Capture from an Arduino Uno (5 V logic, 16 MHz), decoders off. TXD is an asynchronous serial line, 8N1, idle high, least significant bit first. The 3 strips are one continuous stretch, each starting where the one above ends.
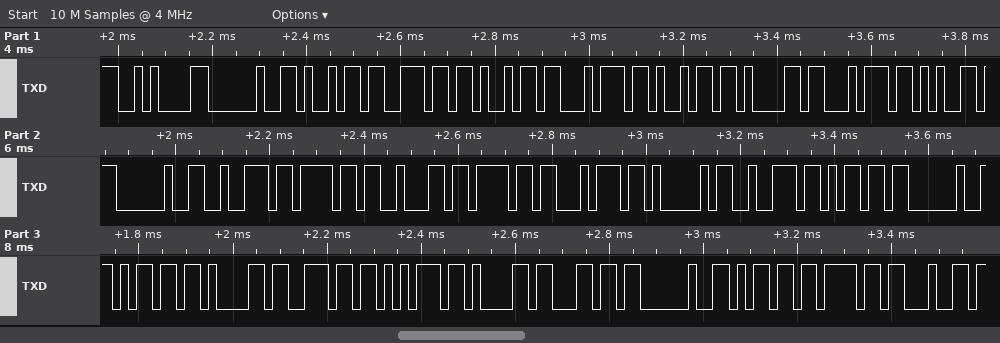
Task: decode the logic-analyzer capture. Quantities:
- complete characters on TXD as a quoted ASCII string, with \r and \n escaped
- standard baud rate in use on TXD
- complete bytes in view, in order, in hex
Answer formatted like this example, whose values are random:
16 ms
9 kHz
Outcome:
"\n initiate robotArm manual mod"
57600 baud
0A 20 69 6E 69 74 69 61 74 65 20 72 6F 62 6F 74 41 72 6D 20 6D 61 6E 75 61 6C 20 6D 6F 64
